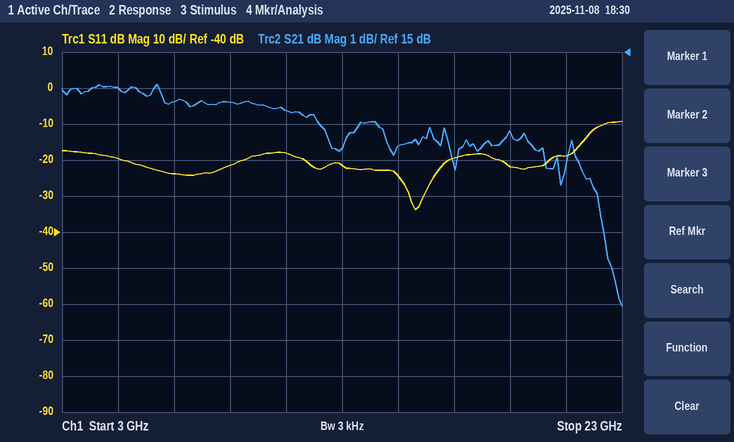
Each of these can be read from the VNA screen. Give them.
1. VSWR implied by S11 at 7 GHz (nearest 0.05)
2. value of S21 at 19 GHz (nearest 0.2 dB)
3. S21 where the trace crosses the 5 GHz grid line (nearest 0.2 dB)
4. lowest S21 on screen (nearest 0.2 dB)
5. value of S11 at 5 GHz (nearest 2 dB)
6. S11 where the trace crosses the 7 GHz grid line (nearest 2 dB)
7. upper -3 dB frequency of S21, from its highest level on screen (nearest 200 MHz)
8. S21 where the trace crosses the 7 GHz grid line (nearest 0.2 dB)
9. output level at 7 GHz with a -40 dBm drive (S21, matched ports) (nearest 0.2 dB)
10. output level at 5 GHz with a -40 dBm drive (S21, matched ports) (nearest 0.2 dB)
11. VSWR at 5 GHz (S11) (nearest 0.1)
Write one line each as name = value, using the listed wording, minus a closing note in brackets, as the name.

VSWR implied by S11 at 7 GHz = 1.15
value of S21 at 19 GHz = 12.8 dB
S21 where the trace crosses the 5 GHz grid line = 14.0 dB
lowest S21 on screen = 8.0 dB
value of S11 at 5 GHz = -20 dB
S11 where the trace crosses the 7 GHz grid line = -24 dB
upper -3 dB frequency of S21, from its highest level on screen = 22.0 GHz
S21 where the trace crosses the 7 GHz grid line = 13.6 dB
output level at 7 GHz with a -40 dBm drive (S21, matched ports) = -26.4 dBm
output level at 5 GHz with a -40 dBm drive (S21, matched ports) = -26.0 dBm
VSWR at 5 GHz (S11) = 1.2
